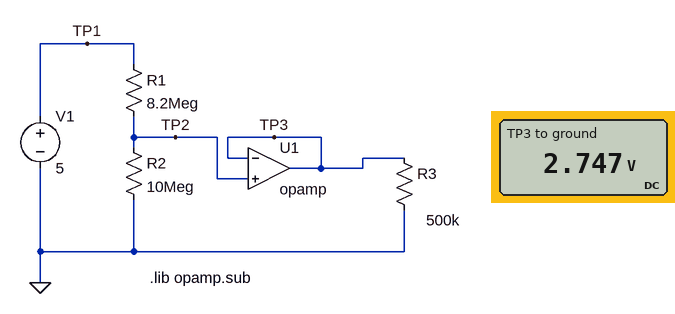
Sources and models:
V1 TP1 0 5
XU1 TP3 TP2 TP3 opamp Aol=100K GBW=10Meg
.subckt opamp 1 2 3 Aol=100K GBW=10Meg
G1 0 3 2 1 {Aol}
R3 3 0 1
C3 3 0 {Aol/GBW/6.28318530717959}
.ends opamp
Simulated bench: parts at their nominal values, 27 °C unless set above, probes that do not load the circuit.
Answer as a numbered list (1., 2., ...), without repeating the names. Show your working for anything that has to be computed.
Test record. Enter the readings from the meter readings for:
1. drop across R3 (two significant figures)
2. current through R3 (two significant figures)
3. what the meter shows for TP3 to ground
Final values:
1. 2.747 V = 2.7 V
2. (2.747 V) / 500 kΩ = 5.5 µA
3. 2.747 V
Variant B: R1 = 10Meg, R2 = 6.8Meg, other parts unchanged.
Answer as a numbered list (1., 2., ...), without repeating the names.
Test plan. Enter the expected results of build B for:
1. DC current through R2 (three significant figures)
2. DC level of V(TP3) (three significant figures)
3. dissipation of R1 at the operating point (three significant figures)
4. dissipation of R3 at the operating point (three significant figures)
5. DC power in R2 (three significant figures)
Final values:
1. 298 nA
2. 2.02 V
3. 886 nW
4. 8.19 µW
5. 602 nW
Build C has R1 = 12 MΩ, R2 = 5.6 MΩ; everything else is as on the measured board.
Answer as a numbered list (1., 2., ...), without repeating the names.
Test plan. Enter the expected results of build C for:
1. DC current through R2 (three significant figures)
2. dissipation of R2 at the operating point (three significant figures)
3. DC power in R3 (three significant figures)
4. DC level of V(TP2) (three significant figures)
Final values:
1. 284 nA
2. 452 nW
3. 5.06 µW
4. 1.59 V
